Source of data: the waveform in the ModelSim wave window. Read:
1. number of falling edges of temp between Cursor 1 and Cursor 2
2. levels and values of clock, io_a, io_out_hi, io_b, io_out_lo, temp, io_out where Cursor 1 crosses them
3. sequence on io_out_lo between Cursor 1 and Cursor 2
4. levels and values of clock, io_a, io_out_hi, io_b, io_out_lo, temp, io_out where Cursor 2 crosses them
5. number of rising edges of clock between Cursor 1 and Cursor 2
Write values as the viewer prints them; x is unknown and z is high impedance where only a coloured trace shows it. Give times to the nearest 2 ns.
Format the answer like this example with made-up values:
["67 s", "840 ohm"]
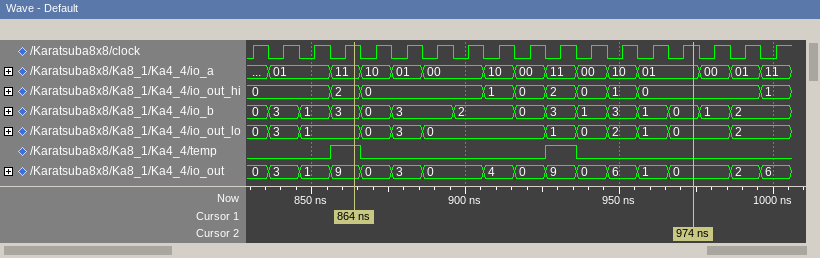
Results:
["2", "clock=1, io_a=11, io_out_hi=2, io_b=3, io_out_lo=1, temp=1, io_out=9", "1, 0, 3, 0, 1, 0, 2, 1, 0", "clock=1, io_a=01, io_out_hi=0, io_b=0, io_out_lo=0, temp=0, io_out=0", "11"]
